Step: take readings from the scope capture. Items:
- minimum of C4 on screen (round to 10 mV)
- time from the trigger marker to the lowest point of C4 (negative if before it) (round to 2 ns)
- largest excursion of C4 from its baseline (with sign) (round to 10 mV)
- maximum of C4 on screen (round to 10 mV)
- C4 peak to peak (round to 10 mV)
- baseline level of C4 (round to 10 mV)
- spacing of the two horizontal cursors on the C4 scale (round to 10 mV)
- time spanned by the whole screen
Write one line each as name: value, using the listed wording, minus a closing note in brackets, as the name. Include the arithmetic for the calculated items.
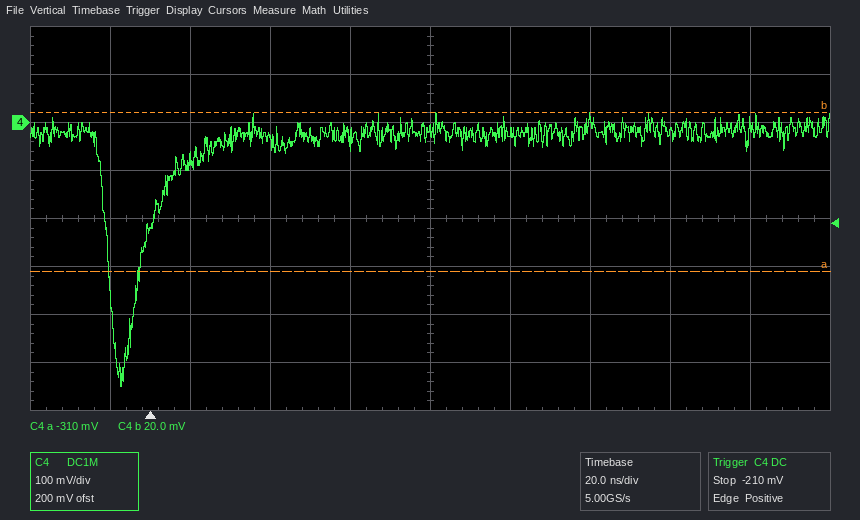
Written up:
minimum of C4 on screen: -550 mV
time from the trigger marker to the lowest point of C4 (negative if before it): -8 ns
largest excursion of C4 from its baseline (with sign): -550 mV − (-20 mV) = -530 mV
maximum of C4 on screen: 20 mV
C4 peak to peak: 20 mV − (-550 mV) = 570 mV
baseline level of C4: -20 mV
spacing of the two horizontal cursors on the C4 scale: 330 mV
time spanned by the whole screen: 200 ns
